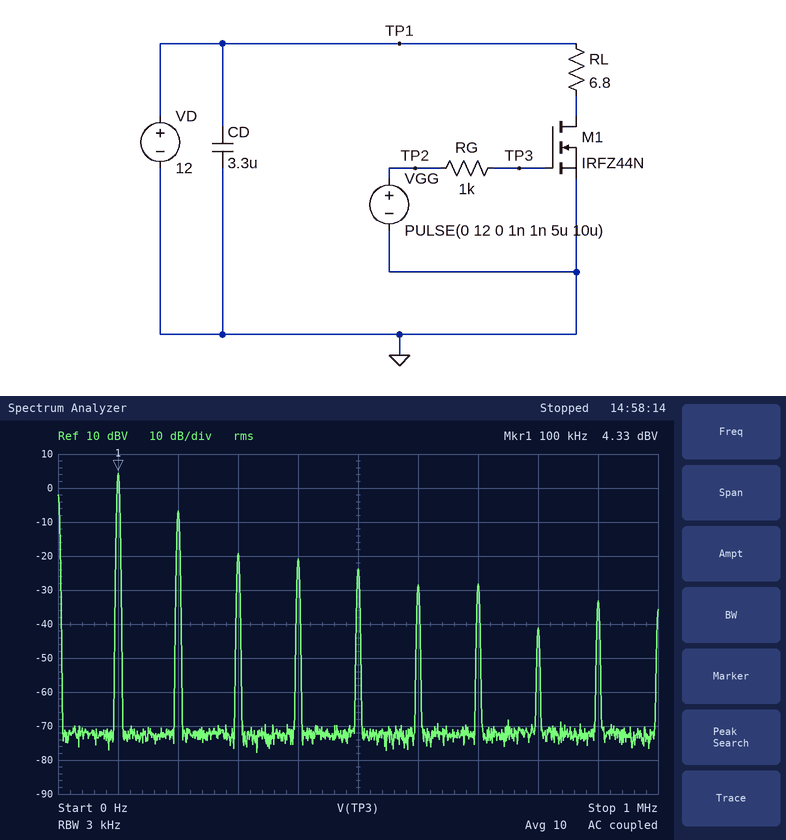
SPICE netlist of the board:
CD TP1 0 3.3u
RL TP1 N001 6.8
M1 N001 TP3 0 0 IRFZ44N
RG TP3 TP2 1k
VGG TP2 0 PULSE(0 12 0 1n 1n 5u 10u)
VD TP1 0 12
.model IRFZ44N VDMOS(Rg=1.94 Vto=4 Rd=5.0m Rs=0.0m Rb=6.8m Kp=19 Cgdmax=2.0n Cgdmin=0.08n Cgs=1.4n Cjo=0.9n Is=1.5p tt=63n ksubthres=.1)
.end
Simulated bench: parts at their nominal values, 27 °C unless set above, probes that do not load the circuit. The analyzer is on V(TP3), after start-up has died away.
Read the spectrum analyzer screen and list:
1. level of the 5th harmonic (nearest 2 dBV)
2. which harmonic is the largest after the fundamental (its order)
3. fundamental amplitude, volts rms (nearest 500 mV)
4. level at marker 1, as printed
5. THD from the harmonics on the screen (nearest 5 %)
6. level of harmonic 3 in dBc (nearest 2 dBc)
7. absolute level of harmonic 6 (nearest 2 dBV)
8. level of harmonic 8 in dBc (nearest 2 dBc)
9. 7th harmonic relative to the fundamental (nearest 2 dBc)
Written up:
-24 dBV
2
1.5 V
4.33 dBV
30 %
-24 dBc
-28 dBV
-46 dBc
-32 dBc
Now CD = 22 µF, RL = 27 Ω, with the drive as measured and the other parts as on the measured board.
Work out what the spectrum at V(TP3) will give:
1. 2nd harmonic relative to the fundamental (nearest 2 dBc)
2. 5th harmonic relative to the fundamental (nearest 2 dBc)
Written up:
-12 dBc
-32 dBc
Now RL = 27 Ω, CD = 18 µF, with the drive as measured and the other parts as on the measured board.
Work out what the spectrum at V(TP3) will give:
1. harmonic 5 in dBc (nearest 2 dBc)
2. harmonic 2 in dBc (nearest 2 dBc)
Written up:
-32 dBc
-12 dBc
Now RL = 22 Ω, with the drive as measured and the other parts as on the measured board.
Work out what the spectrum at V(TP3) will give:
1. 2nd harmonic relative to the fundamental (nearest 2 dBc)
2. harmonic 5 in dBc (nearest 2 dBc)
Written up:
-12 dBc
-30 dBc
